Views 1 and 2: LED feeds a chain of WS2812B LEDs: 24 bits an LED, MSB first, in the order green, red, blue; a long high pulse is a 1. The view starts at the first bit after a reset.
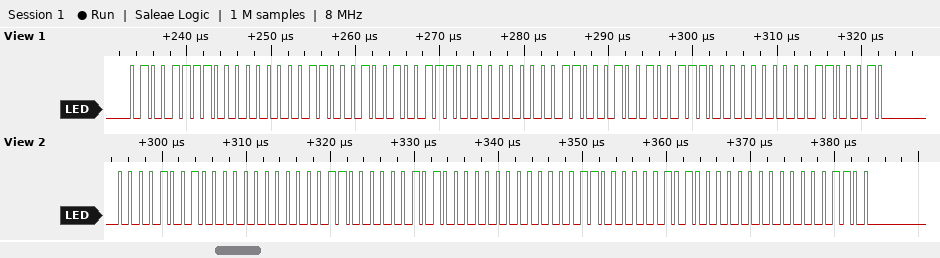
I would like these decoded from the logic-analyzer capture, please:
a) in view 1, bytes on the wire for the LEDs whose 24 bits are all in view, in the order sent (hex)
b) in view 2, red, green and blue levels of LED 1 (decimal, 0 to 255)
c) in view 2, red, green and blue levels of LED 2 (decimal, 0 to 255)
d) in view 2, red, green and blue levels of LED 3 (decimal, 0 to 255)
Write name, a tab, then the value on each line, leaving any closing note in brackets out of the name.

in view 1, bytes on the wire for the LEDs whose 24 bits are all in view, in the order sent	4F 00 62 4E 00 62 4E 00 62
in view 2, red, green and blue levels of LED 1	0, 9, 12
in view 2, red, green and blue levels of LED 2	0, 10, 12
in view 2, red, green and blue levels of LED 3	0, 10, 12
